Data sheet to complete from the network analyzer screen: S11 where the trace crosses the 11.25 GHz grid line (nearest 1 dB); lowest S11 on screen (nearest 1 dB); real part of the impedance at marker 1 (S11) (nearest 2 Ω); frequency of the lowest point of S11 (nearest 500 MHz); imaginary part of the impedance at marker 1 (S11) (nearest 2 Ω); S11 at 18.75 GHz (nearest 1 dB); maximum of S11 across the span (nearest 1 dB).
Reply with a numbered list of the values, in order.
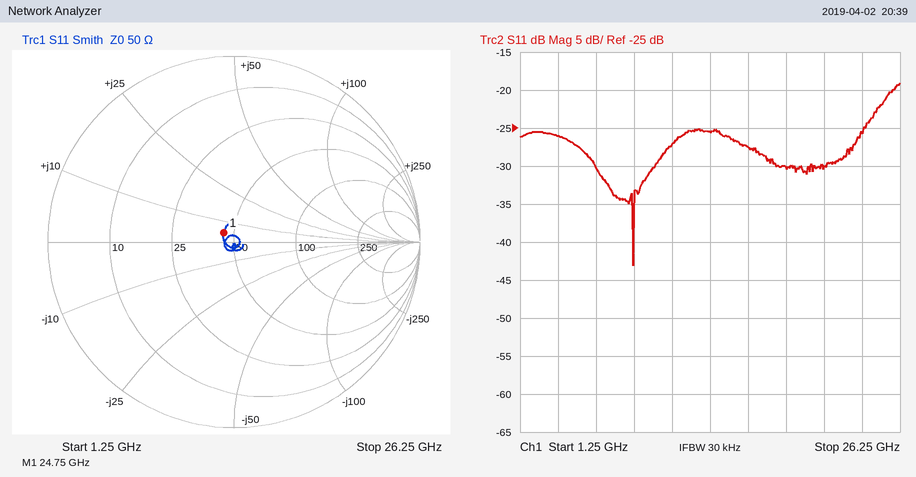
1. -27 dB
2. -43 dB
3. 44 Ω
4. 8.5 GHz
5. +4 Ω
6. -30 dB
7. -19 dB
